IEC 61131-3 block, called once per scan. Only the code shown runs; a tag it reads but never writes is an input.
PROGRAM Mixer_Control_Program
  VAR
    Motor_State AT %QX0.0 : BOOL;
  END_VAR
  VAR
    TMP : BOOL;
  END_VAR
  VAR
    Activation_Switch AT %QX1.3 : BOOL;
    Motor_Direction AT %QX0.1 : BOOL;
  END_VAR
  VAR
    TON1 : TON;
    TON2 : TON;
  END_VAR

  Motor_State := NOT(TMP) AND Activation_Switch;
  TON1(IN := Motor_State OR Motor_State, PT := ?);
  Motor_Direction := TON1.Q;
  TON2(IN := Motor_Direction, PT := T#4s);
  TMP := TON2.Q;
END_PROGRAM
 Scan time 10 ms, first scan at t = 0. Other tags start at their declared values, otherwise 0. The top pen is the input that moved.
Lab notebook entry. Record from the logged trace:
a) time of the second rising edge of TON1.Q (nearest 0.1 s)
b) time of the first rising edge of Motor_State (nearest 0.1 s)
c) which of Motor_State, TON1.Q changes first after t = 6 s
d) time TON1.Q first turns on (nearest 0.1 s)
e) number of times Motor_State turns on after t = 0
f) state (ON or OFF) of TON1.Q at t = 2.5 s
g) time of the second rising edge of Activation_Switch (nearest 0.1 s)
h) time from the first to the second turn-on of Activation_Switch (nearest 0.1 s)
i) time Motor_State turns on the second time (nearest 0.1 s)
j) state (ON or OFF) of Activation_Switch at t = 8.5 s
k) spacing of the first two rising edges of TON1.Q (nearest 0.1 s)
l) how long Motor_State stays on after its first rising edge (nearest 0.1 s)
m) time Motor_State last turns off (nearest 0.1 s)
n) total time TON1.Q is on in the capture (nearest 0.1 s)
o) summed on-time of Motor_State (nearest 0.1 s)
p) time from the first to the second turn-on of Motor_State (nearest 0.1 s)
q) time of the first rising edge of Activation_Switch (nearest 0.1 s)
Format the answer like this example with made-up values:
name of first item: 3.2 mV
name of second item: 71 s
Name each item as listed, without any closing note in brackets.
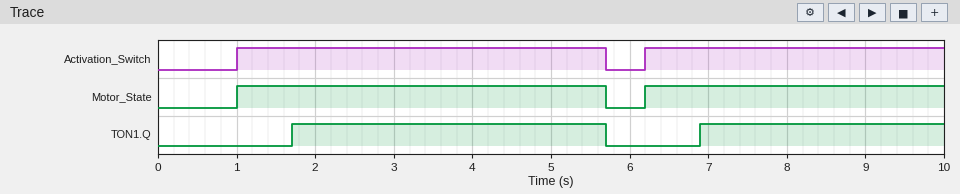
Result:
time of the second rising edge of TON1.Q: 6.9 s
time of the first rising edge of Motor_State: 1.0 s
which of Motor_State, TON1.Q changes first after t = 6 s: Motor_State
time TON1.Q first turns on: 1.7 s
number of times Motor_State turns on after t = 0: 2
state (ON or OFF) of TON1.Q at t = 2.5 s: ON
time of the second rising edge of Activation_Switch: 6.2 s
time from the first to the second turn-on of Activation_Switch: 5.2 s
time Motor_State turns on the second time: 6.2 s
state (ON or OFF) of Activation_Switch at t = 8.5 s: ON
spacing of the first two rising edges of TON1.Q: 5.2 s
how long Motor_State stays on after its first rising edge: 4.7 s
time Motor_State last turns off: 5.7 s
total time TON1.Q is on in the capture: 7.1 s
summed on-time of Motor_State: 8.5 s
time from the first to the second turn-on of Motor_State: 5.2 s
time of the first rising edge of Activation_Switch: 1.0 s
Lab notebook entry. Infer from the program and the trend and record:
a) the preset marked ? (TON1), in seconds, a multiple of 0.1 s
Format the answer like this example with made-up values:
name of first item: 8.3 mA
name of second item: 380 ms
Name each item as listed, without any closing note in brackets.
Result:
the preset marked ? (TON1), in seconds, a multiple of 0.1 s: 0.7 s
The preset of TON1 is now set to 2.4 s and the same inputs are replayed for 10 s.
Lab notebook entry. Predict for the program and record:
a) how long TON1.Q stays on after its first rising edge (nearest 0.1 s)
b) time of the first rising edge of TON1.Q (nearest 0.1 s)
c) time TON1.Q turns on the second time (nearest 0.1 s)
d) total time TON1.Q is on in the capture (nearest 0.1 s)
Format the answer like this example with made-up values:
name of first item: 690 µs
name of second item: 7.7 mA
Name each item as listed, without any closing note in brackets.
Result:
how long TON1.Q stays on after its first rising edge: 2.3 s
time of the first rising edge of TON1.Q: 3.4 s
time TON1.Q turns on the second time: 8.6 s
total time TON1.Q is on in the capture: 3.7 s
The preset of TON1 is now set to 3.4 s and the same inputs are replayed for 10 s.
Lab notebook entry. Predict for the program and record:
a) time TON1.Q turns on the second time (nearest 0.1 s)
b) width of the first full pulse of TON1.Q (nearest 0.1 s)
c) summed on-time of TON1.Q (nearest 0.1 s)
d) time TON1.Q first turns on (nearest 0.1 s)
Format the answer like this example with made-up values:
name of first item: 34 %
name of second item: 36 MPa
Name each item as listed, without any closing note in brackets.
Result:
time TON1.Q turns on the second time: 9.6 s
width of the first full pulse of TON1.Q: 1.3 s
summed on-time of TON1.Q: 1.7 s
time TON1.Q first turns on: 4.4 s
